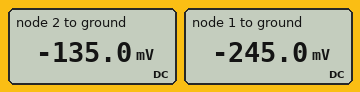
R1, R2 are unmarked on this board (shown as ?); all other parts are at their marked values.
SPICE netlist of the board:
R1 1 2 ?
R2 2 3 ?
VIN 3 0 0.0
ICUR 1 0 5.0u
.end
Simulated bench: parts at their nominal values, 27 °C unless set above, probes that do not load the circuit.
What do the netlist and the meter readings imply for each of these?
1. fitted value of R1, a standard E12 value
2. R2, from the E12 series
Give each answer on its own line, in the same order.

22 kΩ
27 kΩ
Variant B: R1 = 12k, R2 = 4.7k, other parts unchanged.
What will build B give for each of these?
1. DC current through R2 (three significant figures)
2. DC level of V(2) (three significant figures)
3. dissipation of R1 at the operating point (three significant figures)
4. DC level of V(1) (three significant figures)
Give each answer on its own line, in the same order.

5.00 µA
-23.5 mV
300 nW
-83.5 mV
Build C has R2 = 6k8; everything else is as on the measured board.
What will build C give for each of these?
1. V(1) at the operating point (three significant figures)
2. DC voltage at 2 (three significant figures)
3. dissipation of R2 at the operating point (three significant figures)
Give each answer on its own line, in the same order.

-144 mV
-34.0 mV
170 nW
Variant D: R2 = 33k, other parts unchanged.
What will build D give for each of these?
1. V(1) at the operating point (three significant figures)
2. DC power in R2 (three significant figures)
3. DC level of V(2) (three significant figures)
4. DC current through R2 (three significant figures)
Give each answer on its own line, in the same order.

-275 mV
825 nW
-165 mV
5.00 µA
